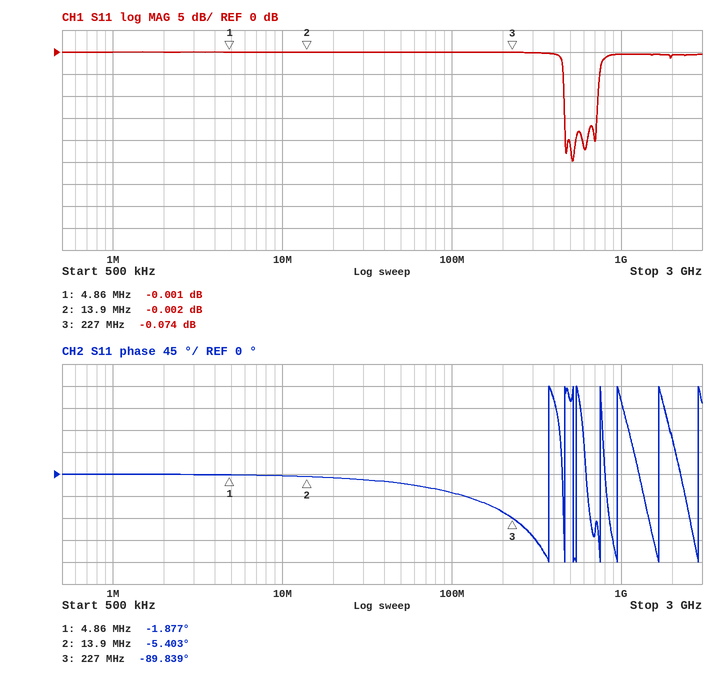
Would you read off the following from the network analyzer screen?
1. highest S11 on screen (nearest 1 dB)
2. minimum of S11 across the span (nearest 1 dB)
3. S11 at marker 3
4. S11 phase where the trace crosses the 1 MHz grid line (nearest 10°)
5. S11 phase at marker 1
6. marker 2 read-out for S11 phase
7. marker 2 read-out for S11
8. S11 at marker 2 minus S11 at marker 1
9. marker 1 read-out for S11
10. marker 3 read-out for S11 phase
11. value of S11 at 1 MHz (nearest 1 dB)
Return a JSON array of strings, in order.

["0 dB", "-25 dB", "-0.074 dB", "0°", "-1.877°", "-5.403°", "-0.002 dB", "-0.001 dB", "-0.001 dB", "-89.839°", "0 dB"]
